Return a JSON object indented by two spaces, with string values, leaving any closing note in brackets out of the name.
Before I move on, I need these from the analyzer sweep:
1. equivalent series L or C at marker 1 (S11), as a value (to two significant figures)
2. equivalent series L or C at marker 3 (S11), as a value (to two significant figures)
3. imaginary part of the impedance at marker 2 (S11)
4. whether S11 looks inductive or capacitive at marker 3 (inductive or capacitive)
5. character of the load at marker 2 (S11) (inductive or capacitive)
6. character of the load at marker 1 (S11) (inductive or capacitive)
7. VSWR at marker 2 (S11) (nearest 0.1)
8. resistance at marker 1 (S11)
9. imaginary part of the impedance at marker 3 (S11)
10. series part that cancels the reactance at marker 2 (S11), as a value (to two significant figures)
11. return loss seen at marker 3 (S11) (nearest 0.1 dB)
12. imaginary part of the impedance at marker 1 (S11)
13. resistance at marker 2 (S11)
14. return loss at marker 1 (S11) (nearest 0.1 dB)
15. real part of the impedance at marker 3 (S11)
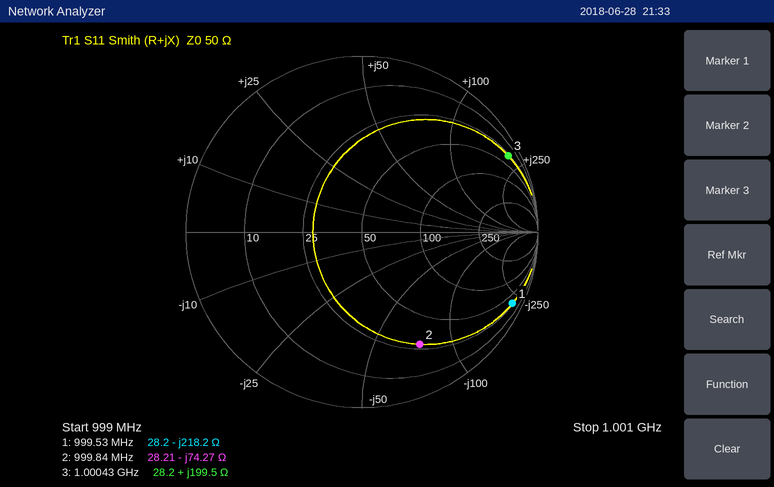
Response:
{
  "equivalent series L or C at marker 1 (S11), as a value": "730 fF",
  "equivalent series L or C at marker 3 (S11), as a value": "32 nH",
  "imaginary part of the impedance at marker 2": "-74.27 Ω",
  "whether S11 looks inductive or capacitive at marker 3": "inductive",
  "character of the load at marker 2 (S11)": "capacitive",
  "character of the load at marker 1 (S11)": "capacitive",
  "VSWR at marker 2 (S11)": "6.1",
  "resistance at marker 1": "28.2 Ω",
  "imaginary part of the impedance at marker 3": "+199.5 Ω",
  "series part that cancels the reactance at marker 2 (S11), as a value": "12 nH",
  "return loss seen at marker 3 (S11)": "0.6 dB",
  "imaginary part of the impedance at marker 1": "-218.2 Ω",
  "resistance at marker 2": "28.21 Ω",
  "return loss at marker 1 (S11)": "0.5 dB",
  "real part of the impedance at marker 3": "28.2 Ω"
}
